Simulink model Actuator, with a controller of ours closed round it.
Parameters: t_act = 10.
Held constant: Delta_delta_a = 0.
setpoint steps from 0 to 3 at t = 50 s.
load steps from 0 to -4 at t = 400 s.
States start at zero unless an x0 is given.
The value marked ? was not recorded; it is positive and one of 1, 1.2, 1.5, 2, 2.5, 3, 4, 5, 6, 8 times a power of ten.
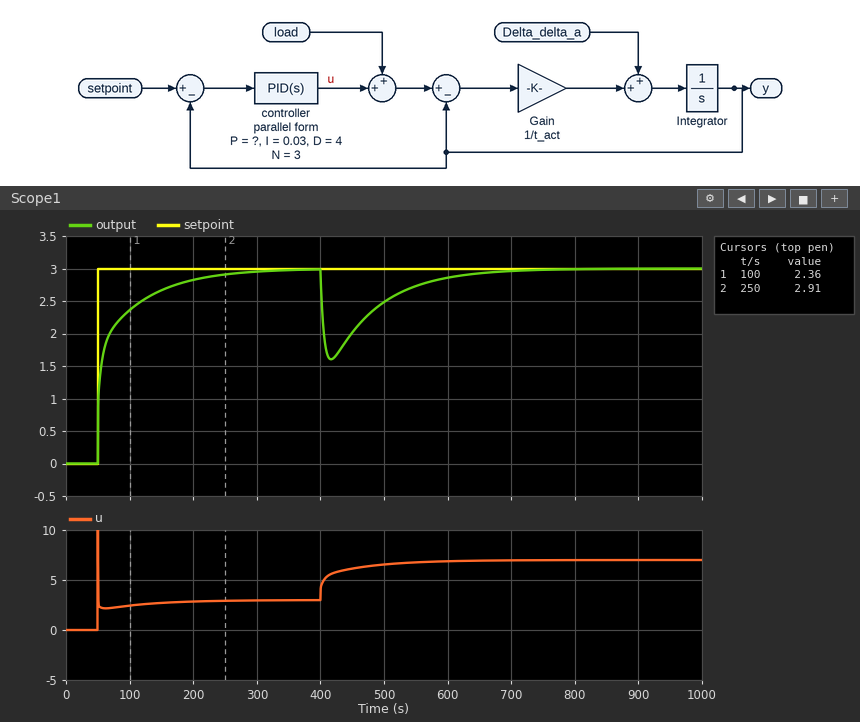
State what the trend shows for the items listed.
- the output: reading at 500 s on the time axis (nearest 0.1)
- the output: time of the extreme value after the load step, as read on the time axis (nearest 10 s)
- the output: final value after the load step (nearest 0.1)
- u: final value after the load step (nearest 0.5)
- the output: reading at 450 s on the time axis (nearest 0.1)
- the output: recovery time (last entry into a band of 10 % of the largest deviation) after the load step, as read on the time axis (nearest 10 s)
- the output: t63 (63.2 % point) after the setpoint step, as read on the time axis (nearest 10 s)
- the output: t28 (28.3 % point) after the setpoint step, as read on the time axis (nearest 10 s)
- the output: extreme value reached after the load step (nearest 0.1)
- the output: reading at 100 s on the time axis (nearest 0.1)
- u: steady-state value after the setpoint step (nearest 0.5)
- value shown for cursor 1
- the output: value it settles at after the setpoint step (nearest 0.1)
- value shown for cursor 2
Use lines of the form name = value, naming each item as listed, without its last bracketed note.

the output: reading at 500 s on the time axis = 2.5
the output: time of the extreme value after the load step, as read on the time axis = 420 s
the output: final value after the load step = 3.0
u: final value after the load step = 7.0
the output: reading at 450 s on the time axis = 2.0
the output: recovery time (last entry into a band of 10 % of the largest deviation) after the load step, as read on the time axis = 600 s
the output: t63 (63.2 % point) after the setpoint step, as read on the time axis = 60 s
the output: t28 (28.3 % point) after the setpoint step, as read on the time axis = 50 s
the output: extreme value reached after the load step = 1.6
the output: reading at 100 s on the time axis = 2.4
u: steady-state value after the setpoint step = 3.0
value shown for cursor 1 = 2.36
the output: value it settles at after the setpoint step = 3.0
value shown for cursor 2 = 2.91
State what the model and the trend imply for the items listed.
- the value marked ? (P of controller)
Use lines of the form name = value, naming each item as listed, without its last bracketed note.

the value marked ? = 1.5
